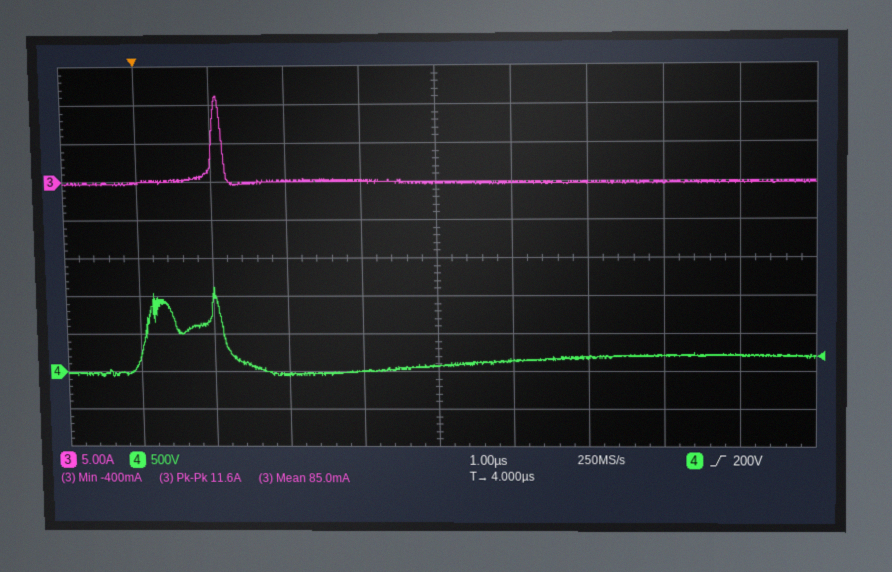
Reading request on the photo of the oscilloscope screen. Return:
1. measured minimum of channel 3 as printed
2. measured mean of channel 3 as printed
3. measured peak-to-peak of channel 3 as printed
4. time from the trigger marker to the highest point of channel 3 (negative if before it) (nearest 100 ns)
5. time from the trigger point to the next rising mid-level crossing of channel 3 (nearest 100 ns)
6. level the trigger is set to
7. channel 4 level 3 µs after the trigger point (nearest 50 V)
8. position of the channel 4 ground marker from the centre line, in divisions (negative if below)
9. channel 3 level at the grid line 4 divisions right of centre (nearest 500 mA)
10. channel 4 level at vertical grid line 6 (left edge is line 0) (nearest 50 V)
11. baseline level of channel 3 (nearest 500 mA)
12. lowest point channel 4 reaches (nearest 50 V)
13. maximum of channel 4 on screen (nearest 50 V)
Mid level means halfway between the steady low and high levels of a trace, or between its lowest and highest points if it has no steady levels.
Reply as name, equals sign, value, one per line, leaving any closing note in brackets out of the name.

measured minimum of channel 3 as printed = -400 mA
measured mean of channel 3 as printed = 85.0 mA
measured peak-to-peak of channel 3 as printed = 11.6 A
time from the trigger marker to the highest point of channel 3 (negative if before it) = +1.1 µs
time from the trigger point to the next rising mid-level crossing of channel 3 = 1.0 µs
level the trigger is set to = 200 V
channel 4 level 3 µs after the trigger point = 0 V
position of the channel 4 ground marker from the centre line, in divisions = -3.0 div
channel 3 level at the grid line 4 divisions right of centre = 0.0 A
channel 4 level at vertical grid line 6 (left edge is line 0) = 150 V
baseline level of channel 3 = 0.0 A
lowest point channel 4 reaches = -50 V
maximum of channel 4 on screen = 1.10 kV
